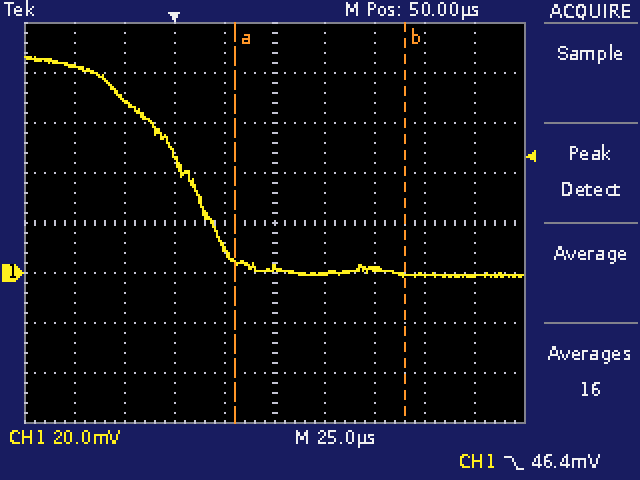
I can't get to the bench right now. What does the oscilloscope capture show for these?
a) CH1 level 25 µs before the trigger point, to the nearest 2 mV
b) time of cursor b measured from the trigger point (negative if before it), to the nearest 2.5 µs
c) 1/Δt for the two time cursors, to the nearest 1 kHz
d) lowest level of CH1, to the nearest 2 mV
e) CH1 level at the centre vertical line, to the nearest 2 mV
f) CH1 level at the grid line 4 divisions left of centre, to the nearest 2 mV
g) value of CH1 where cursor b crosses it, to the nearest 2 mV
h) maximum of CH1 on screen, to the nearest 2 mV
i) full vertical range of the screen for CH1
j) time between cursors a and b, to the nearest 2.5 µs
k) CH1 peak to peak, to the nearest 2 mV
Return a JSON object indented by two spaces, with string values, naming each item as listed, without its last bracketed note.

{
  "CH1 level 25 µs before the trigger point, to the nearest 2 mV": "70 mV",
  "time of cursor b measured from the trigger point (negative if before it), to the nearest 2.5 µs": "+115.0 µs",
  "1/Δt for the two time cursors, to the nearest 1 kHz": "12 kHz",
  "lowest level of CH1, to the nearest 2 mV": "-2 mV",
  "CH1 level at the centre vertical line, to the nearest 2 mV": "2 mV",
  "CH1 level at the grid line 4 divisions left of centre, to the nearest 2 mV": "82 mV",
  "value of CH1 where cursor b crosses it, to the nearest 2 mV": "0 mV",
  "maximum of CH1 on screen, to the nearest 2 mV": "86 mV",
  "full vertical range of the screen for CH1": "160 mV",
  "time between cursors a and b, to the nearest 2.5 µs": "85.0 µs",
  "CH1 peak to peak, to the nearest 2 mV": "88 mV"
}
